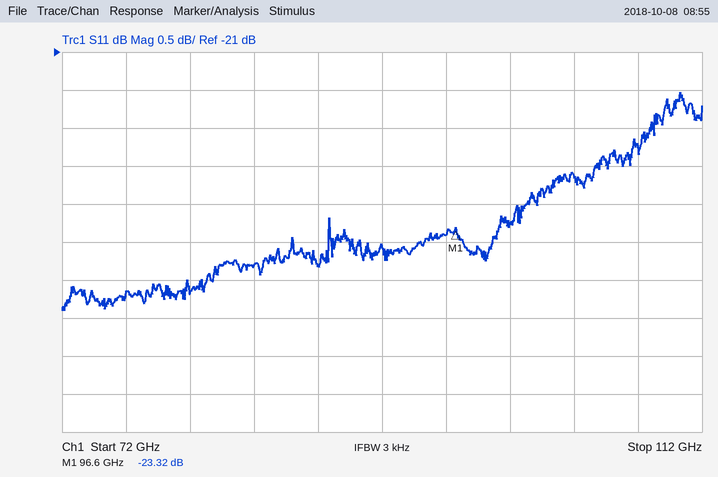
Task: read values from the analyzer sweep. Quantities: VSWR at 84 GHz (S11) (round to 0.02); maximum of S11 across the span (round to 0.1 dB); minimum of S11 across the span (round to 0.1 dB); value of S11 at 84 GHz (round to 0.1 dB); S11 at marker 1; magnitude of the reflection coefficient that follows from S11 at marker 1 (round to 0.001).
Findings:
1.14
-21.5 dB
-24.4 dB
-23.8 dB
-23.32 dB
0.068
